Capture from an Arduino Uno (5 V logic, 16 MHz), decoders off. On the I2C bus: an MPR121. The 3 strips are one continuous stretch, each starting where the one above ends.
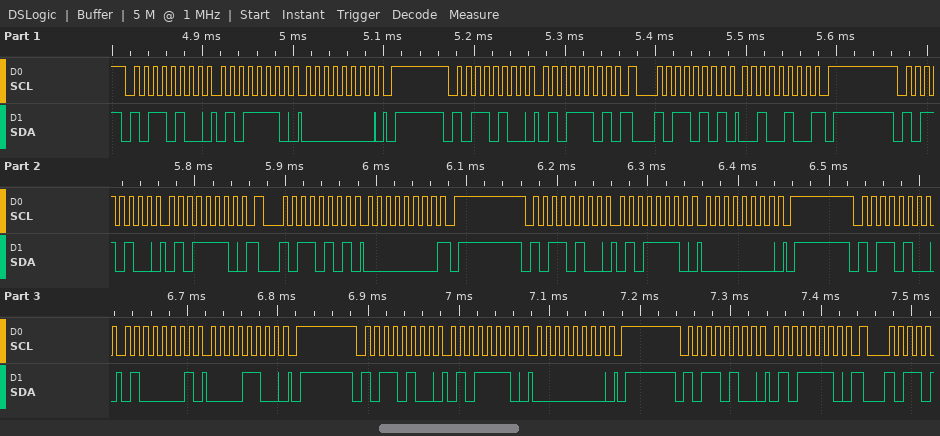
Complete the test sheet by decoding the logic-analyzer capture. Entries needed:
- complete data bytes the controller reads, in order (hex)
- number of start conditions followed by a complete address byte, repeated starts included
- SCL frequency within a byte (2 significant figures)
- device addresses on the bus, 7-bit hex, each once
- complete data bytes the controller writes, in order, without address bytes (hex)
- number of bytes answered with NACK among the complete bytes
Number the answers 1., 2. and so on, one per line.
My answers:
1. 24 00
2. 9
3. 100 kHz
4. 0x5A
5. 5E 00 5D 5E 5E 00 41 0C 5E 00 5E
6. 2
